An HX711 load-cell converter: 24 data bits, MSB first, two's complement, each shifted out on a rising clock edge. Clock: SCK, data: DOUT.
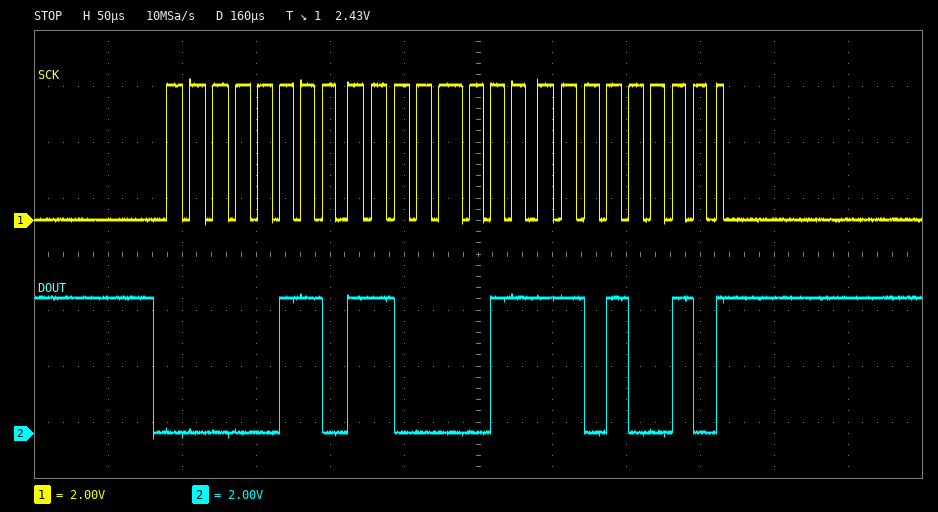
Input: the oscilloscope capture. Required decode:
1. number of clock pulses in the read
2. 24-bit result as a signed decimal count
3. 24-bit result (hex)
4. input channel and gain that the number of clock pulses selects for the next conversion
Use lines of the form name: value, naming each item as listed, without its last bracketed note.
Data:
number of clock pulses in the read: 25
24-bit result as a signed decimal count: 443346
24-bit result: 0x06C3D2
input channel and gain that the number of clock pulses selects for the next conversion: channel A, gain 128
